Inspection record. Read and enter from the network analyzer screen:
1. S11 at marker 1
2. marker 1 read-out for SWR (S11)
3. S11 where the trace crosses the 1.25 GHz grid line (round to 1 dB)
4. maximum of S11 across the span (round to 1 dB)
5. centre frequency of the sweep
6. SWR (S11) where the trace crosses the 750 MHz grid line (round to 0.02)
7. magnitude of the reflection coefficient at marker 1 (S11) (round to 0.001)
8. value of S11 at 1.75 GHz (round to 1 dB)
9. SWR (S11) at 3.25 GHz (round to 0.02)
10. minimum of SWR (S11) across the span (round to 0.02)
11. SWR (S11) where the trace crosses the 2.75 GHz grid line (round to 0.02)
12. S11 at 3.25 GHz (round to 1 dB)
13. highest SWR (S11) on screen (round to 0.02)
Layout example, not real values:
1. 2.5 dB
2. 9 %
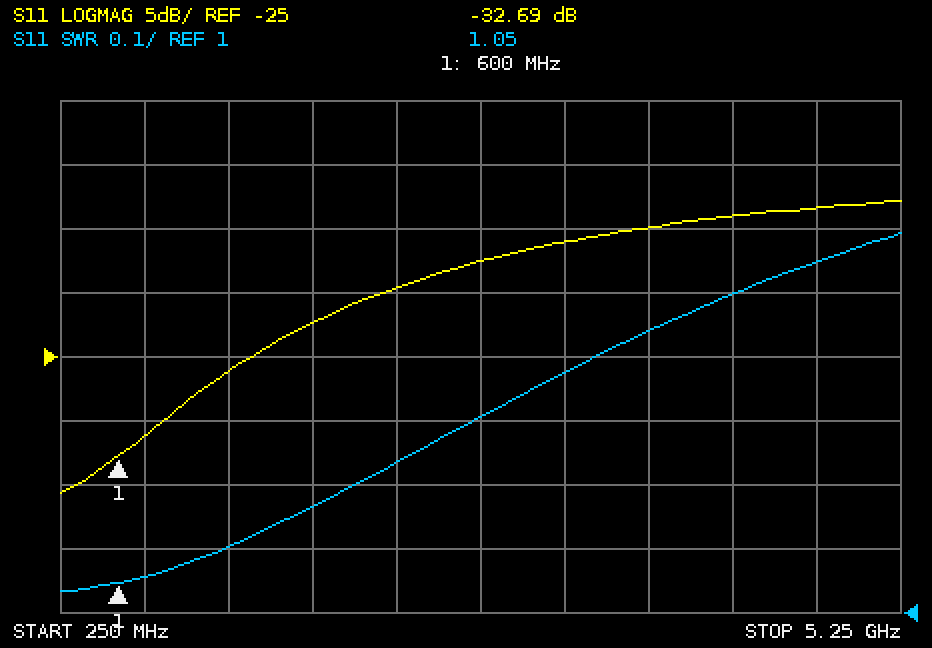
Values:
1. -32.69 dB
2. 1.05
3. -26 dB
4. -13 dB
5. 2.75 GHz
6. 1.06
7. 0.023
8. -22 dB
9. 1.38
10. 1.04
11. 1.30
12. -16 dB
13. 1.60
